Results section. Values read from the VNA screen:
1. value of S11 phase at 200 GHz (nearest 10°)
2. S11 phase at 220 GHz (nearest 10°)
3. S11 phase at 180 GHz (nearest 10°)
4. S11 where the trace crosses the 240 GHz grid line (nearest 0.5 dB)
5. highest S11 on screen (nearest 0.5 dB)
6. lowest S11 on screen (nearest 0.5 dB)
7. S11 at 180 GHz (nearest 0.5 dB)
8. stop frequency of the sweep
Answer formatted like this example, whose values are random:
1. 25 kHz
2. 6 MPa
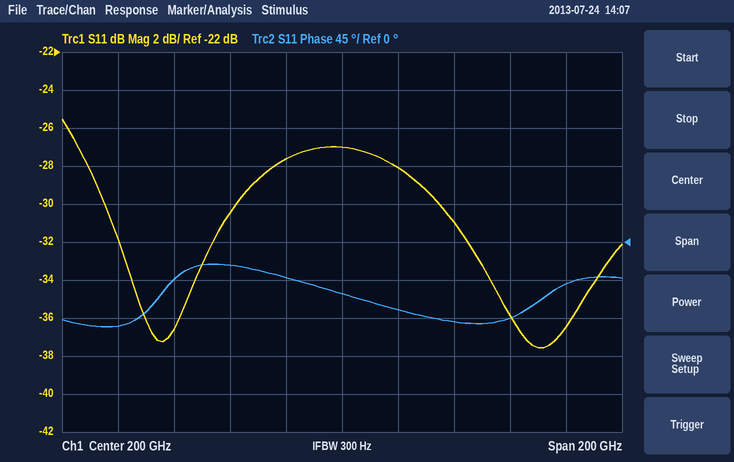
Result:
1. -60°
2. -80°
3. -40°
4. -31.0 dB
5. -25.5 dB
6. -37.5 dB
7. -27.5 dB
8. 300 GHz
